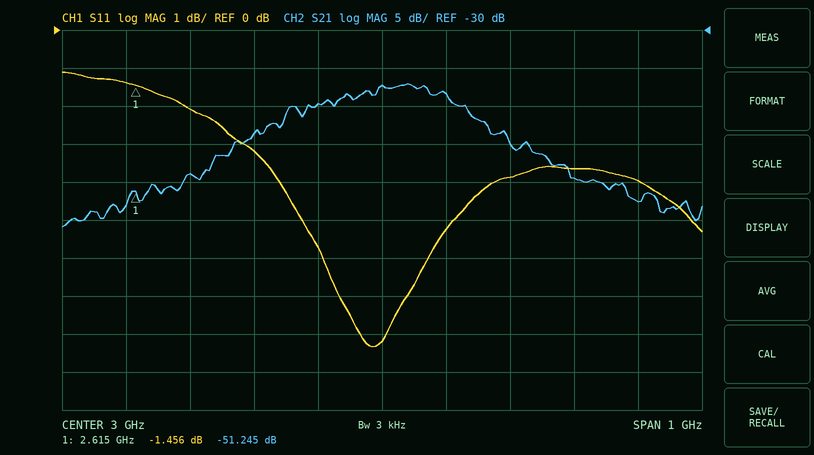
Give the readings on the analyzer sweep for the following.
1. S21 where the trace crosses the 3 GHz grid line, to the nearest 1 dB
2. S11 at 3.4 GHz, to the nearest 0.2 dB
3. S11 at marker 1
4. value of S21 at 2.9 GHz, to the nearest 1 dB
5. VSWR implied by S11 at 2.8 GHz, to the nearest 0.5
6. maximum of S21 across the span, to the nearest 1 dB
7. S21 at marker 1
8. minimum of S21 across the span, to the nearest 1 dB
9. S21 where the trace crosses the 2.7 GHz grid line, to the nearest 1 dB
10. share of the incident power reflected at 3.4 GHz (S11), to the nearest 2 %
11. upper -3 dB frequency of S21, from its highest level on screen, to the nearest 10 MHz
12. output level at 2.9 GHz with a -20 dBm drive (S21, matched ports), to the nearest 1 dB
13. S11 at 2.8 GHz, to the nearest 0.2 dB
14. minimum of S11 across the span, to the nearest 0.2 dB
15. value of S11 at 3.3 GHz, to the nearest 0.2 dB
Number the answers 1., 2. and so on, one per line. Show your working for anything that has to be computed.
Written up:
1. -37 dB
2. -4.0 dB
3. -1.456 dB
4. -40 dB
5. |Γ| = 10^(-3.2/20) = 0.6918; VSWR = (1 + 0.6918)/(1 − 0.6918) ≈ 5.5
6. -37 dB
7. -51.245 dB
8. -56 dB
9. -49 dB
10. 10^(-4/10) ≈ 40 %
11. 3.13 GHz
12. -20 dBm + (-40 dB) = -60 dBm
13. -3.2 dB
14. -8.4 dB
15. -3.6 dB
